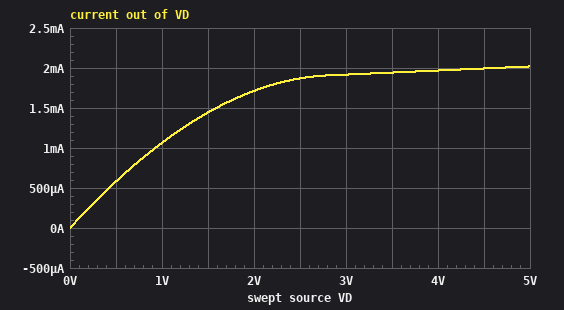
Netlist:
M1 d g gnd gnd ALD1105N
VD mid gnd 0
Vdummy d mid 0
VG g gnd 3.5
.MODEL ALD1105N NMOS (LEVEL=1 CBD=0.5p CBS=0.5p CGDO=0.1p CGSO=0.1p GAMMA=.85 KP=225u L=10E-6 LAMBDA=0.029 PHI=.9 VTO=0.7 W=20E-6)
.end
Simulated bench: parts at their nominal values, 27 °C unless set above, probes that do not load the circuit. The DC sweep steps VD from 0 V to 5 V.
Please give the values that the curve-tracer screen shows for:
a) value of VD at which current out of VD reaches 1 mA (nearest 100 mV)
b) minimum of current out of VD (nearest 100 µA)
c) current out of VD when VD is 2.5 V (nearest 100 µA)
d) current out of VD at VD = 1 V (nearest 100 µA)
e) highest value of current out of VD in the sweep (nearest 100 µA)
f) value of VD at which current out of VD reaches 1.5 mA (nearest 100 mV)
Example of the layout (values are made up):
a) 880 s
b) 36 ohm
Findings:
a) 900 mV
b) 0 A
c) 1.9 mA
d) 1.1 mA
e) 2.0 mA
f) 1.6 V
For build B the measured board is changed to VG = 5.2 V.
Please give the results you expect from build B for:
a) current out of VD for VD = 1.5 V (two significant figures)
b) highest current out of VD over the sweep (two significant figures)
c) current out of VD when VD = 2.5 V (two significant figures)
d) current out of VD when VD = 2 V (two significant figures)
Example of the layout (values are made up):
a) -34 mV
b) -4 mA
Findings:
a) 2.6 mA
b) 5.2 mA
c) 3.9 mA
d) 3.3 mA
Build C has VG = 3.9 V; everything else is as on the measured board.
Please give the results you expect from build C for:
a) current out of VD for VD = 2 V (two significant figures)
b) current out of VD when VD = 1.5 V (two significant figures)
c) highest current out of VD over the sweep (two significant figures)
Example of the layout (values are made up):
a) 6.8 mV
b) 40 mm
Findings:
a) 2.1 mA
b) 1.7 mA
c) 2.6 mA
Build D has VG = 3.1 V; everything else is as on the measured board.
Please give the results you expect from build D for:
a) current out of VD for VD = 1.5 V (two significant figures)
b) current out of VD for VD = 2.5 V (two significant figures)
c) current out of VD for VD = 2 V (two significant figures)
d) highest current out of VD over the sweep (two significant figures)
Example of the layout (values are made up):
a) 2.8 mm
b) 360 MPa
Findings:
a) 1.2 mA
b) 1.4 mA
c) 1.3 mA
d) 1.5 mA
